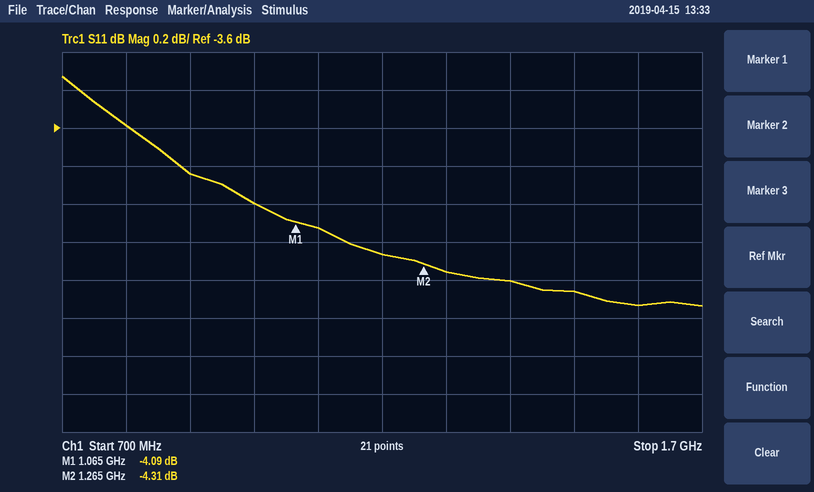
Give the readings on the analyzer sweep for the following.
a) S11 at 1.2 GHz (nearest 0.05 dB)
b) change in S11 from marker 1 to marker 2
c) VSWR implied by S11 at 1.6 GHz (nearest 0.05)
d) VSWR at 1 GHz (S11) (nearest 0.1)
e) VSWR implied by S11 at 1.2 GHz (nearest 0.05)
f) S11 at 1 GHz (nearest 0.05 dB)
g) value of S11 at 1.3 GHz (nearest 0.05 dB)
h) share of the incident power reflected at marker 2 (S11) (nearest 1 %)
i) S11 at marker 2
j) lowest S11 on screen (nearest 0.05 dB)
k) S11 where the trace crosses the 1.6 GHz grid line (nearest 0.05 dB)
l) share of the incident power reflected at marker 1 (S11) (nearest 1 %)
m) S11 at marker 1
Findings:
-4.25 dB
-0.22 dB
3.90
4.4
4.15
-4.00 dB
-4.35 dB
37 %
-4.31 dB
-4.55 dB
-4.55 dB
39 %
-4.09 dB
